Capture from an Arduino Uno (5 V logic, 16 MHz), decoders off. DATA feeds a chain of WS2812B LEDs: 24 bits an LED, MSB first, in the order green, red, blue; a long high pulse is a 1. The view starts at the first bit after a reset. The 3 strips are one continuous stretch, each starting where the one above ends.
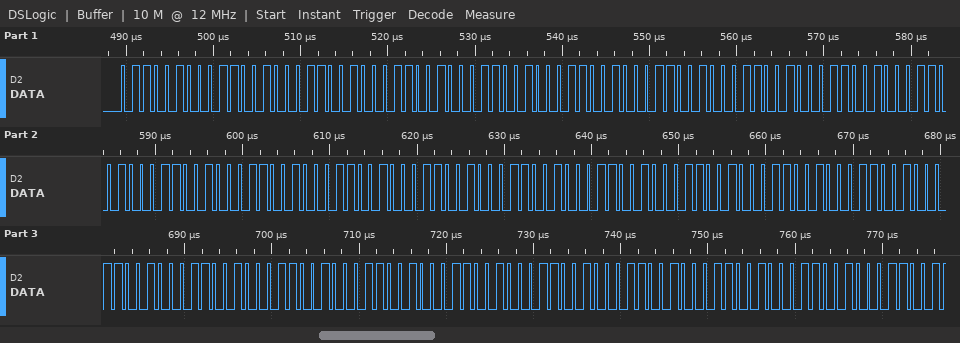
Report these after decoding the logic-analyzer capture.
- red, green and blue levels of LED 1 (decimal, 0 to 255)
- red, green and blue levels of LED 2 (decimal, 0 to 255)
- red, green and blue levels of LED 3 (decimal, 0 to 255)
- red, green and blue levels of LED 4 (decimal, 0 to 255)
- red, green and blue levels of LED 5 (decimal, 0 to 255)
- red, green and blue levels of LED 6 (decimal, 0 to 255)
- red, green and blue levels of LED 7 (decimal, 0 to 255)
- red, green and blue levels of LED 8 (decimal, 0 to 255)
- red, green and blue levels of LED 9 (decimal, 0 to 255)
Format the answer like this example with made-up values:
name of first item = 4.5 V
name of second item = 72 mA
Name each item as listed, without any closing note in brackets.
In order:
red, green and blue levels of LED 1 = 100, 100, 100
red, green and blue levels of LED 2 = 100, 100, 100
red, green and blue levels of LED 3 = 100, 100, 100
red, green and blue levels of LED 4 = 100, 100, 100
red, green and blue levels of LED 5 = 100, 100, 100
red, green and blue levels of LED 6 = 100, 100, 100
red, green and blue levels of LED 7 = 100, 100, 100
red, green and blue levels of LED 8 = 100, 100, 100
red, green and blue levels of LED 9 = 100, 100, 100
